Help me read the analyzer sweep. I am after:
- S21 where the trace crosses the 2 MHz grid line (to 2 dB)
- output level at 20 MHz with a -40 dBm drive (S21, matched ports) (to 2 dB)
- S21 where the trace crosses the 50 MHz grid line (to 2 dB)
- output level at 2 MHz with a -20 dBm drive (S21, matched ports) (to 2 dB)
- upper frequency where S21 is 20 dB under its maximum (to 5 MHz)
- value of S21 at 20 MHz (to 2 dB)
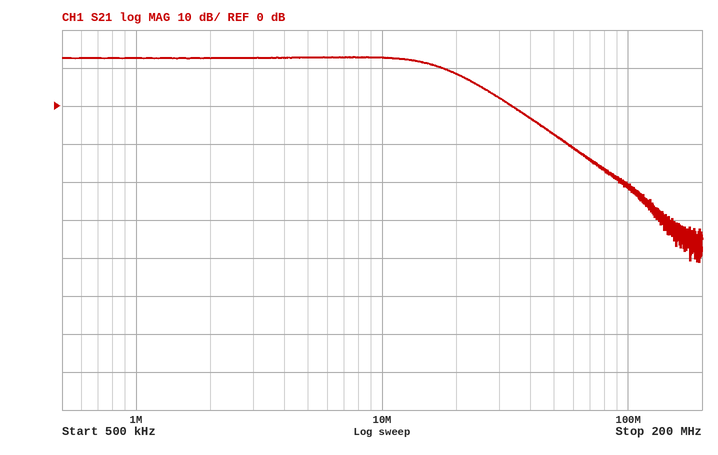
12 dB
-32 dBm
-8 dB
-8 dBm
50 MHz
8 dB
